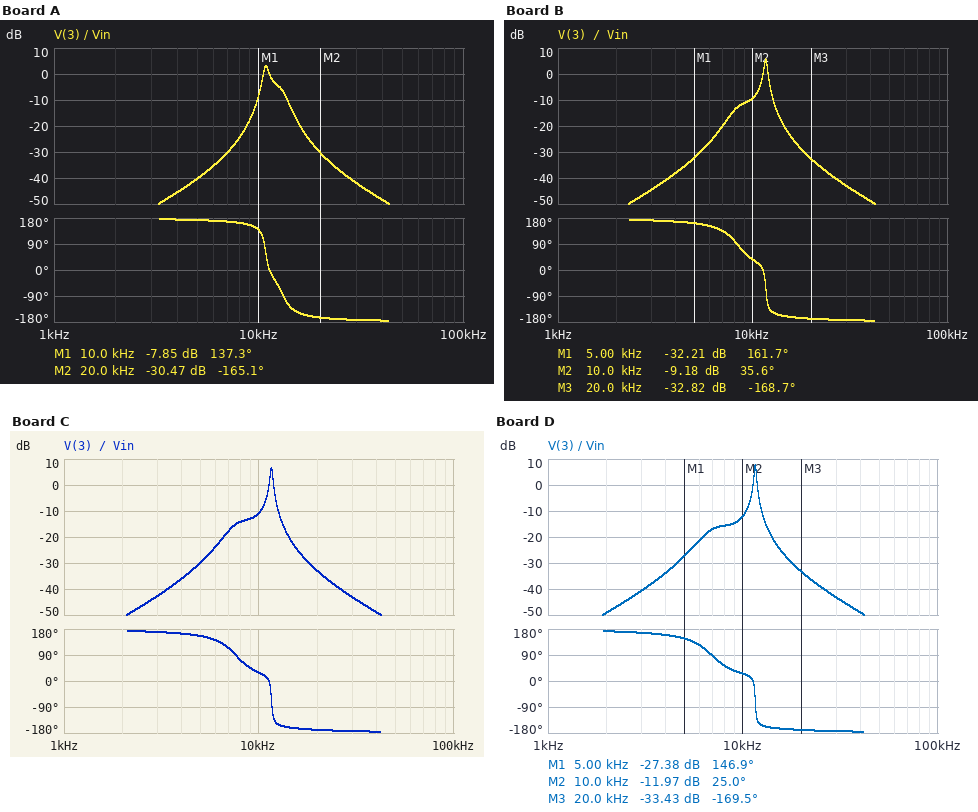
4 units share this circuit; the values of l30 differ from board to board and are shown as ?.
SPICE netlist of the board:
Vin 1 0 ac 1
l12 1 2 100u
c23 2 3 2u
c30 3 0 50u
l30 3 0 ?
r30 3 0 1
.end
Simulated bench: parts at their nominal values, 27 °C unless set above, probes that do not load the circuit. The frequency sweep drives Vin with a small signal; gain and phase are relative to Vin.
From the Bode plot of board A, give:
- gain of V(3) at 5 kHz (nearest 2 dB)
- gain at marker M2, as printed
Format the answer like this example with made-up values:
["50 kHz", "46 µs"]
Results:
["-40 dB", "-30.47 dB"]
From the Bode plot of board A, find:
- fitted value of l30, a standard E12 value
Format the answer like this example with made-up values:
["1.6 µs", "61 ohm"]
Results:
["3.3 µH"]
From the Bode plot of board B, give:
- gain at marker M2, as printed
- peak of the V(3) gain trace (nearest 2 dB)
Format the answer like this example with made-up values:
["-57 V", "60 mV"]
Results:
["-9.18 dB", "6 dB"]
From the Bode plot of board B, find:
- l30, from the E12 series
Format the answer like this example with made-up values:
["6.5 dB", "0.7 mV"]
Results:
["6.8 µH"]
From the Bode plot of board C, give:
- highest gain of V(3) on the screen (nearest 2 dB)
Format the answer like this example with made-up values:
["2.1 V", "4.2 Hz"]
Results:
["6 dB"]
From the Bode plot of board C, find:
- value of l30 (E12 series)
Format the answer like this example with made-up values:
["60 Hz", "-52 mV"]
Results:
["8.2 µH"]
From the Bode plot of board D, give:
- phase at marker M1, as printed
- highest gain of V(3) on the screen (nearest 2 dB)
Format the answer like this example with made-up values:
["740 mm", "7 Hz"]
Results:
["146.9 deg", "8 dB"]
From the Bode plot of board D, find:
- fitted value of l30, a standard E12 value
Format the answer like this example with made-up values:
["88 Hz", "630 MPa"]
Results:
["10 µH"]
